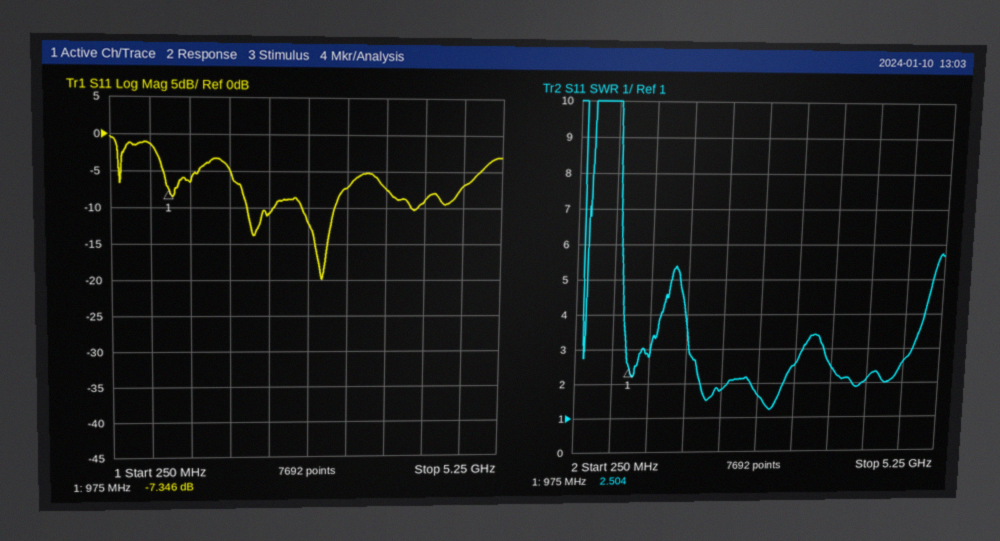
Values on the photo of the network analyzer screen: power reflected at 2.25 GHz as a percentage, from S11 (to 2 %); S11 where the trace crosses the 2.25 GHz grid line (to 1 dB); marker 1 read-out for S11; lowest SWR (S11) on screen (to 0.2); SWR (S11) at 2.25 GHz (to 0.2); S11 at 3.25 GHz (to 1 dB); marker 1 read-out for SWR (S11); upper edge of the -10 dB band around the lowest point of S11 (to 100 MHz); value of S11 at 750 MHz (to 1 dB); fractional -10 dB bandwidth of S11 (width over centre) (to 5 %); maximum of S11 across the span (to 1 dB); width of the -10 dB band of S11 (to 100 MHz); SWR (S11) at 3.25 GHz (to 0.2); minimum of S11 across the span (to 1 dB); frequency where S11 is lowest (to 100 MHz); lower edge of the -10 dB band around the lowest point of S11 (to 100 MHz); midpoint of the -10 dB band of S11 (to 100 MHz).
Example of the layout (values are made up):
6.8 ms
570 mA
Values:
8 %
-11 dB
-7.346 dB
1.2
1.8
-7 dB
2.504
3.1 GHz
-1 dB
15 %
0 dB
400 MHz
2.6
-20 dB
2.9 GHz
2.7 GHz
2.9 GHz
